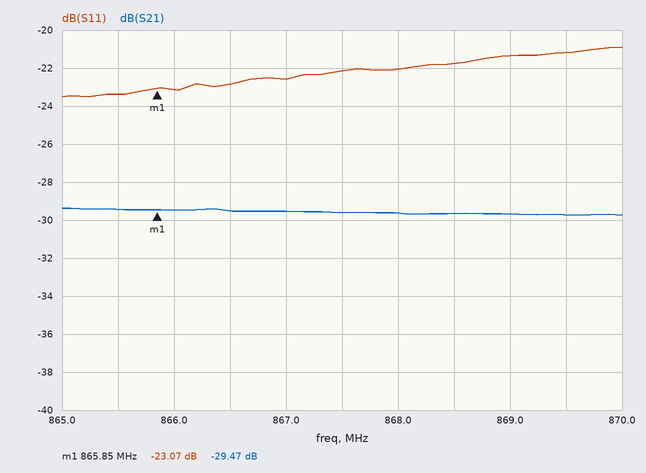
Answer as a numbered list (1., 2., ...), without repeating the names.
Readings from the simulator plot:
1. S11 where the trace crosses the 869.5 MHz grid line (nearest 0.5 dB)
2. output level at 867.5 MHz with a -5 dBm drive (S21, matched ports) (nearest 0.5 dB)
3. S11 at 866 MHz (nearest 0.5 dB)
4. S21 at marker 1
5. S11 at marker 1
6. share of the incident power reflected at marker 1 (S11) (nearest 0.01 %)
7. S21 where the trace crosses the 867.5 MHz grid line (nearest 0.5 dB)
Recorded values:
1. -21.0 dB
2. -34.5 dBm
3. -23.0 dB
4. -29.47 dB
5. -23.07 dB
6. 0.49 %
7. -29.5 dB
